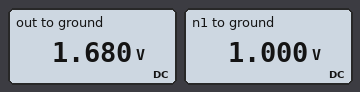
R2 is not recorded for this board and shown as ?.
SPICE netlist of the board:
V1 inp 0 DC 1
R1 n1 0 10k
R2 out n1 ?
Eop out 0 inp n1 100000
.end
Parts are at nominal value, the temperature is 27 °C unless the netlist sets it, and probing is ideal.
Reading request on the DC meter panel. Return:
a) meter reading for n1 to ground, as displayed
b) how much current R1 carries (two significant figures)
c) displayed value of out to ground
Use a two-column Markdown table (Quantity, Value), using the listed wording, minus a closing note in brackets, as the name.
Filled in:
| Quantity | Value |
|---|---|
| meter reading for n1 to ground, as displayed | 1.000 V |
| how much current R1 carries | 100 µA |
| displayed value of out to ground | 1.680 V |
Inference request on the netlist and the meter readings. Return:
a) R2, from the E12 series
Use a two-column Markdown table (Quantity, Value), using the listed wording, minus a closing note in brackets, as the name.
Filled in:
| Quantity | Value |
|---|---|
| R2, from the E12 series | 6.8 kΩ |
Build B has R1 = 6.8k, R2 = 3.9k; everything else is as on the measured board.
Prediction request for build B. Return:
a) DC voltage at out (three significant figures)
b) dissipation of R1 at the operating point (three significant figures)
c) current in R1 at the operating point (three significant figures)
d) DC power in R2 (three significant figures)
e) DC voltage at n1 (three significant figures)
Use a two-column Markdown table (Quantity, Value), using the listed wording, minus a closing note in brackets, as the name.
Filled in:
| Quantity | Value |
|---|---|
| DC voltage at out | 1.57 V |
| dissipation of R1 at the operating point | 147 µW |
| current in R1 at the operating point | 147 µA |
| DC power in R2 | 84.3 µW |
| DC voltage at n1 | 1.00 V |
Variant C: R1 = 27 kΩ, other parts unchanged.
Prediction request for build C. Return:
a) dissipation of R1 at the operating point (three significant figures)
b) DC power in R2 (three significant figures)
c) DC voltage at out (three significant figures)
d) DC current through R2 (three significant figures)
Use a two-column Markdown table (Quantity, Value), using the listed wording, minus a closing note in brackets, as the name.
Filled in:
| Quantity | Value |
|---|---|
| dissipation of R1 at the operating point | 37.0 µW |
| DC power in R2 | 9.33 µW |
| DC voltage at out | 1.25 V |
| DC current through R2 | 37.0 µA |
